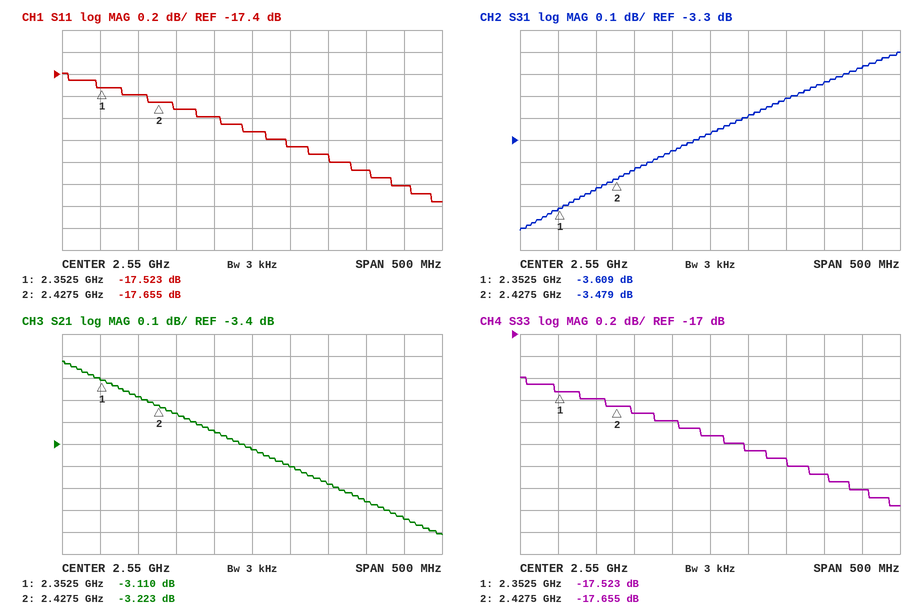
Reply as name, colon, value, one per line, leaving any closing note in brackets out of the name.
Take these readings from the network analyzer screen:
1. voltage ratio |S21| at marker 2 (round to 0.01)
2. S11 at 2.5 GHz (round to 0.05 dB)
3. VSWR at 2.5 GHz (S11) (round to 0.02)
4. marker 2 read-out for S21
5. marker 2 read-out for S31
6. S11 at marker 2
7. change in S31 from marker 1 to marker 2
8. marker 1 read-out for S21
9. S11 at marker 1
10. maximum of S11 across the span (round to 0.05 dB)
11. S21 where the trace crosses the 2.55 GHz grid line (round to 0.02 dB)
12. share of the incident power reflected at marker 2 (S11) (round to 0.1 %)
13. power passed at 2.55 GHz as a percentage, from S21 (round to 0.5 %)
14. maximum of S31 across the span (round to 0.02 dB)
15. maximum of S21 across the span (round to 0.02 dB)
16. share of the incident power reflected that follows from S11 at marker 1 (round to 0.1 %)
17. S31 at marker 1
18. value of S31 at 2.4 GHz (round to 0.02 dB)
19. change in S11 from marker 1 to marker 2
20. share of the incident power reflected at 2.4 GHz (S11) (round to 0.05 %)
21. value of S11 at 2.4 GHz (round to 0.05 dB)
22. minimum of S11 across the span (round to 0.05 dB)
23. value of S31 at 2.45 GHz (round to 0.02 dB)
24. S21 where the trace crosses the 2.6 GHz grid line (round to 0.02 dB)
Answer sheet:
voltage ratio |S21| at marker 2: 0.69
S11 at 2.5 GHz: -17.80 dB
VSWR at 2.5 GHz (S11): 1.30
marker 2 read-out for S21: -3.223 dB
marker 2 read-out for S31: -3.479 dB
S11 at marker 2: -17.655 dB
change in S31 from marker 1 to marker 2: 0.130 dB
marker 1 read-out for S21: -3.110 dB
S11 at marker 1: -17.523 dB
maximum of S11 across the span: -17.40 dB
S21 where the trace crosses the 2.55 GHz grid line: -3.42 dB
share of the incident power reflected at marker 2 (S11): 1.7 %
power passed at 2.55 GHz as a percentage, from S21: 45.5 %
maximum of S31 across the span: -2.90 dB
maximum of S21 across the span: -3.02 dB
share of the incident power reflected that follows from S11 at marker 1: 1.8 %
S31 at marker 1: -3.609 dB
value of S31 at 2.4 GHz: -3.52 dB
change in S11 from marker 1 to marker 2: -0.132 dB
share of the incident power reflected at 2.4 GHz (S11): 1.75 %
value of S11 at 2.4 GHz: -17.60 dB
minimum of S11 across the span: -18.55 dB
value of S31 at 2.45 GHz: -3.44 dB
S21 where the trace crosses the 2.6 GHz grid line: -3.50 dB
